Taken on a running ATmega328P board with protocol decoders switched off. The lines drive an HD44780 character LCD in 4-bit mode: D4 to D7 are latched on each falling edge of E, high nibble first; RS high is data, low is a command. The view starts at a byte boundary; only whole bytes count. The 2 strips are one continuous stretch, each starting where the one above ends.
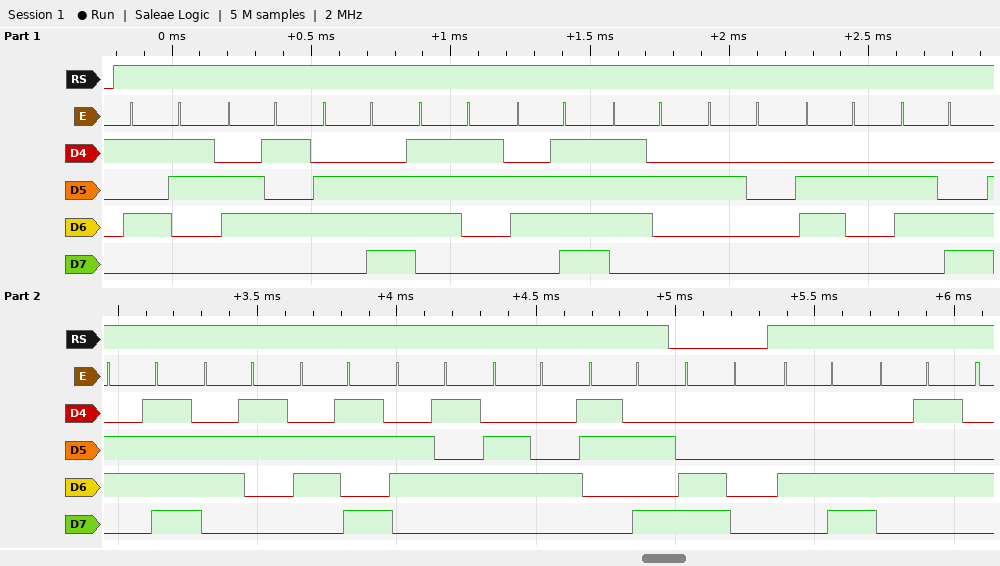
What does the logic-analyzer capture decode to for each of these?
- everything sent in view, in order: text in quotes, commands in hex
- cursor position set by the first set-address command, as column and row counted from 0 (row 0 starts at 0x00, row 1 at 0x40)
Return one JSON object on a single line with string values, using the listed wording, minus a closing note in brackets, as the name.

{"everything sent in view, in order: text in quotes, commands in hex": "\"Sensor blocked:\" 0xC0 \"LE\"", "cursor position set by the first set-address command, as column and row counted from 0": "column 0, row 1"}
